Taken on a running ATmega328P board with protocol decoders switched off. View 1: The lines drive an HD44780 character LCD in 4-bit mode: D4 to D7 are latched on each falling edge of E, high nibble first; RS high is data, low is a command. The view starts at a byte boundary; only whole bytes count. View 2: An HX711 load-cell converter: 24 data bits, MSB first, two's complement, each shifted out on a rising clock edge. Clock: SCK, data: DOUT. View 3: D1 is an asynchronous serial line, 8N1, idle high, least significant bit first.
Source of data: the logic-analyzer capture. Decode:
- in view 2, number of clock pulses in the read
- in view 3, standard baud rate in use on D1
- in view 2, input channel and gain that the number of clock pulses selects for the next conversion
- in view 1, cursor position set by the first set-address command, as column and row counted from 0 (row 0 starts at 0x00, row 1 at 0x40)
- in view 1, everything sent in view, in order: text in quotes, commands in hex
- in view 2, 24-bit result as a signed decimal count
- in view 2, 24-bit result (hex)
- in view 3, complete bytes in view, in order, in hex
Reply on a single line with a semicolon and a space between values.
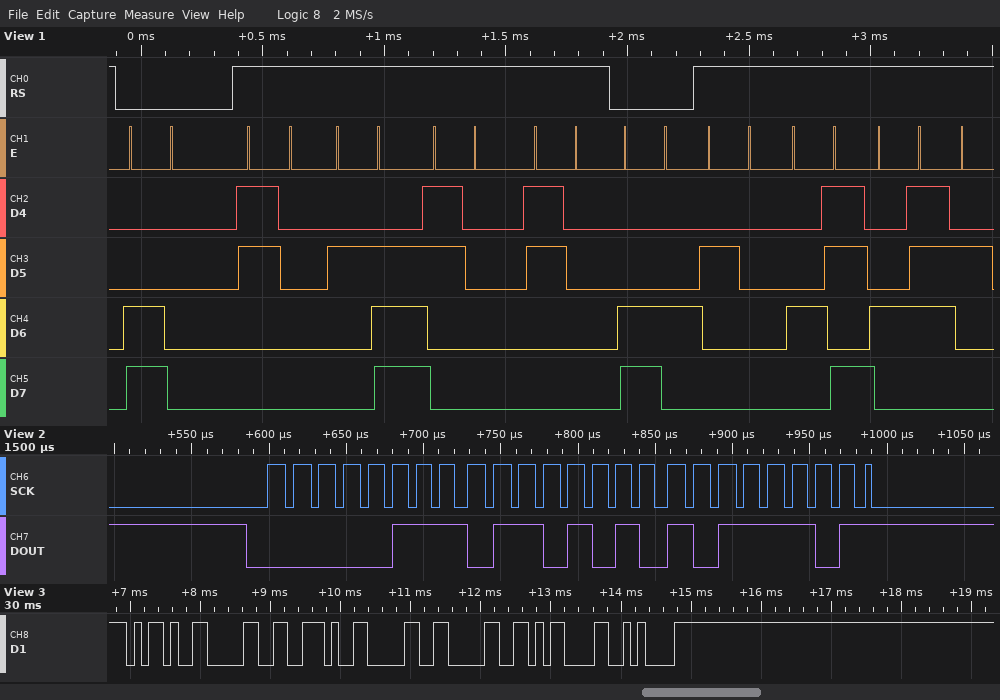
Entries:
25; 9600 baud; channel A, gain 128; column 0, row 1; 0xC0 "0.00" 0xC4 " KG"; 486077; 0x076ABD; 2D 30 2E 30 30 0D 0A
